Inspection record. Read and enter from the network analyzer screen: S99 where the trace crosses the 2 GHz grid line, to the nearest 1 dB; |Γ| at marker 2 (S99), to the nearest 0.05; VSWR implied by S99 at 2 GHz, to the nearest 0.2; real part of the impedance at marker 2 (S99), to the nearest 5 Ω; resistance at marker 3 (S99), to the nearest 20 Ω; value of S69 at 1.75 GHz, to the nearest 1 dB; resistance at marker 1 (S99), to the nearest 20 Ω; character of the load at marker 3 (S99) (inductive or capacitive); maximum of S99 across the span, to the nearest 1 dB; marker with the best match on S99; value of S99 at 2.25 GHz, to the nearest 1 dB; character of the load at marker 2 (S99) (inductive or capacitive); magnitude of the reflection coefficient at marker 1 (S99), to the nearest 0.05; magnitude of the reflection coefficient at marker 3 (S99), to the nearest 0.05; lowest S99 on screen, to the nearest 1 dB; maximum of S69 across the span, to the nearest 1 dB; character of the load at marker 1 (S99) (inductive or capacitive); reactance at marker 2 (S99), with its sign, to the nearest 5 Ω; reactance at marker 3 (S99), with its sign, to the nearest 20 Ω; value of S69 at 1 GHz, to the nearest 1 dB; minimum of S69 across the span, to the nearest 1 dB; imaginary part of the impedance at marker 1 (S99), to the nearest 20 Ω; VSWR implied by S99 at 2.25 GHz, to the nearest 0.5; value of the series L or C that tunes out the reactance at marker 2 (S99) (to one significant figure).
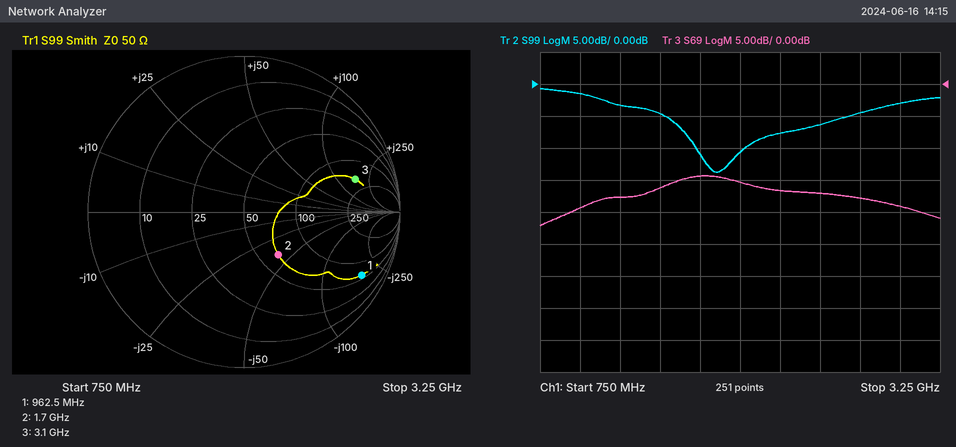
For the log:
-11 dB
0.35
1.8
65 Ω
180 Ω
-14 dB
60 Ω
inductive
-1 dB
marker 2
-8 dB
capacitive
0.85
0.75
-14 dB
-14 dB
capacitive
-40 Ω
+160 Ω
-19 dB
-22 dB
-180 Ω
2.5
4 nH
